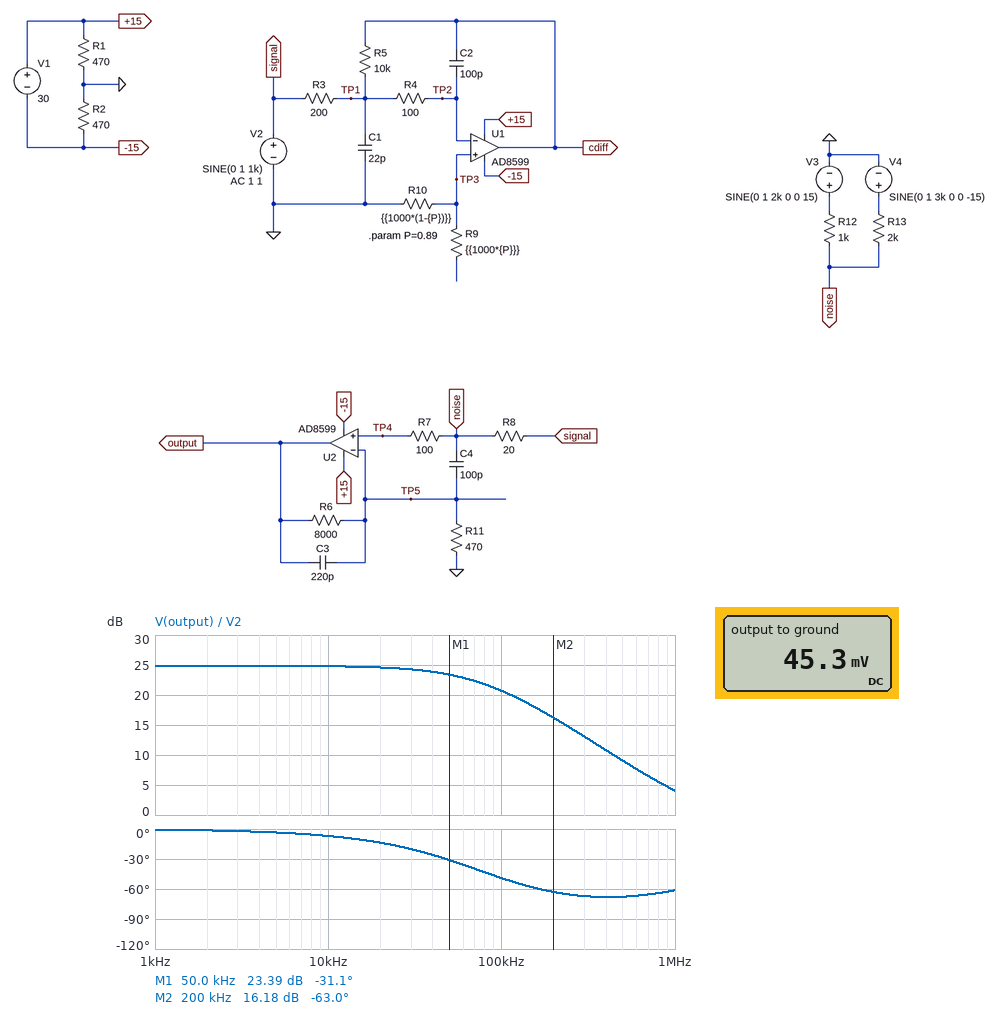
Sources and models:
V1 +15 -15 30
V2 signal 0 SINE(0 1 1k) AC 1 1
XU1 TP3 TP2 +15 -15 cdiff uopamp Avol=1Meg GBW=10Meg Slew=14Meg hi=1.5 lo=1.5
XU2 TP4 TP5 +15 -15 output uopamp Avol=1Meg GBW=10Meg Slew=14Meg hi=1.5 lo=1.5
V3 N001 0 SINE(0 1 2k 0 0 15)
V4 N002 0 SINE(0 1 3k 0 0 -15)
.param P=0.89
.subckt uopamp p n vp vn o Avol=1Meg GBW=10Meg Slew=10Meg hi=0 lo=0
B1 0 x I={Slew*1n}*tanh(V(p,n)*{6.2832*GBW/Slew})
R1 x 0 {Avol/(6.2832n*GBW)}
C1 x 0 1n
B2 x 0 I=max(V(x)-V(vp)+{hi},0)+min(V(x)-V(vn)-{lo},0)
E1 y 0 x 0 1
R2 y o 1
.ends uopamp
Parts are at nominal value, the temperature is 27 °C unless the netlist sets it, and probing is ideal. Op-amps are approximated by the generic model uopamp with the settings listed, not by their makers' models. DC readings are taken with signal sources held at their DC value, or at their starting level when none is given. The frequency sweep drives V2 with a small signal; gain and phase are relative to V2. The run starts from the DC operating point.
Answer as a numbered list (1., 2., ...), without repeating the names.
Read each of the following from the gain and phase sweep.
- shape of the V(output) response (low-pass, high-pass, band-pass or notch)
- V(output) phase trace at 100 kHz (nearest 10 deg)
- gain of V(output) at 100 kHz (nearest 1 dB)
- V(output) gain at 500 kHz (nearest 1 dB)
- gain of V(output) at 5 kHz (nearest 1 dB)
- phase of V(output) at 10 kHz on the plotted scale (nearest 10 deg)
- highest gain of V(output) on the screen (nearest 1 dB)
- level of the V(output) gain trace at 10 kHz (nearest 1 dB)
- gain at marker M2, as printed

1. low-pass
2. -50 deg
3. 21 dB
4. 9 dB
5. 25 dB
6. -10 deg
7. 25 dB
8. 25 dB
9. 16.18 dB
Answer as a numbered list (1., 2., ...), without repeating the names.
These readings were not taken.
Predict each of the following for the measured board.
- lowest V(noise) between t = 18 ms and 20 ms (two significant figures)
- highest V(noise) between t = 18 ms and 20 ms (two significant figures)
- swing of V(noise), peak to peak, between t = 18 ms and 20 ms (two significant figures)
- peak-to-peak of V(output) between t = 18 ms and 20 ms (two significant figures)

1. -970 mV
2. 960 mV
3. 1.9 V
4. 27 V
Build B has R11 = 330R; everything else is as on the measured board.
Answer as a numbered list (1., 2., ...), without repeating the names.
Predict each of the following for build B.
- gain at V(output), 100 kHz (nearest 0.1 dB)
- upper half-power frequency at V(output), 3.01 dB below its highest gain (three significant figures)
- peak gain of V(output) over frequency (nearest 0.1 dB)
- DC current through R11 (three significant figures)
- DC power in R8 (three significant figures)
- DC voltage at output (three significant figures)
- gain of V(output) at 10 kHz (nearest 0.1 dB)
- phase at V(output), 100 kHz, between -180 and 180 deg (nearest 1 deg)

1. 23.3 dB
2. 74.4 kHz
3. 27.8 dB
4. 7.61 µA
5. 316 nW
6. 63.4 mV
7. 27.7 dB
8. -52 deg
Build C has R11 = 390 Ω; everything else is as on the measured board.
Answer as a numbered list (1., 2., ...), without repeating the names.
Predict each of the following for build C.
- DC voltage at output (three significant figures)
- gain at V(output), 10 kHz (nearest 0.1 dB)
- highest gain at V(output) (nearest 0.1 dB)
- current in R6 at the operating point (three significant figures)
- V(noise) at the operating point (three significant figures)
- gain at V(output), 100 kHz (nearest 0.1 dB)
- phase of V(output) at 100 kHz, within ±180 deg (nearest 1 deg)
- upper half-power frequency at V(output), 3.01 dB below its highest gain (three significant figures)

1. 54.1 mV
2. 26.3 dB
3. 26.4 dB
4. 6.44 µA
5. 2.51 mV
6. 22.1 dB
7. -50 deg
8. 76.5 kHz
